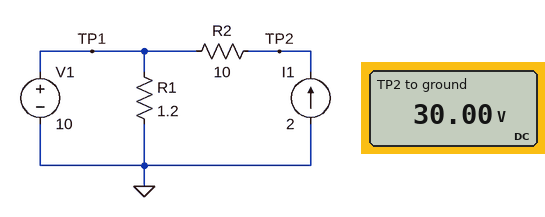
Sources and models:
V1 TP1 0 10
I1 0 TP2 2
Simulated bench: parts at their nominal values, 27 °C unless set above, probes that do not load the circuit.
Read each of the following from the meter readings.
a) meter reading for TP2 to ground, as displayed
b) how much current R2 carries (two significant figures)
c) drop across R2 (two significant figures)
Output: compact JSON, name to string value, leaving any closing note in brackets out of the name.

{"meter reading for TP2 to ground, as displayed": "30.00 V", "how much current R2 carries": "2.0 A", "drop across R2": "20 V"}
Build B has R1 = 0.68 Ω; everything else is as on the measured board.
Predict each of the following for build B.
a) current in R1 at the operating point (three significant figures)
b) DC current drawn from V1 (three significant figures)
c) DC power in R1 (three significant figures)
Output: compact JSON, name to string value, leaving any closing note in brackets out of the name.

{"current in R1 at the operating point": "14.7 A", "DC current drawn from V1": "12.7 A", "DC power in R1": "147 W"}
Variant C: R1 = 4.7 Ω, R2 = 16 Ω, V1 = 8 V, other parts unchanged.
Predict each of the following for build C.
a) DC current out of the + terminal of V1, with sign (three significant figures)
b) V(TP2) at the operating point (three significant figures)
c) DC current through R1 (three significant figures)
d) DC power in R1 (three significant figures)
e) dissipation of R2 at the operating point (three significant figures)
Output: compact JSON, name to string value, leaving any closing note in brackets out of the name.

{"DC current out of the + terminal of V1, with sign": "-298 mA", "V(TP2) at the operating point": "40.0 V", "DC current through R1": "1.70 A", "DC power in R1": "13.6 W", "dissipation of R2 at the operating point": "64.0 W"}
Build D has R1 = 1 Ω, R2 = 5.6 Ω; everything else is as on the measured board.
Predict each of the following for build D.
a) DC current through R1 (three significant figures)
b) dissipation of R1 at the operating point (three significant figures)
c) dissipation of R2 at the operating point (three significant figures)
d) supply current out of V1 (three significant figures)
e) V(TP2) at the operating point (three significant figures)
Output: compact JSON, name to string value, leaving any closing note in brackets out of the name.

{"DC current through R1": "10.0 A", "dissipation of R1 at the operating point": "100 W", "dissipation of R2 at the operating point": "22.4 W", "supply current out of V1": "8.00 A", "V(TP2) at the operating point": "21.2 V"}
